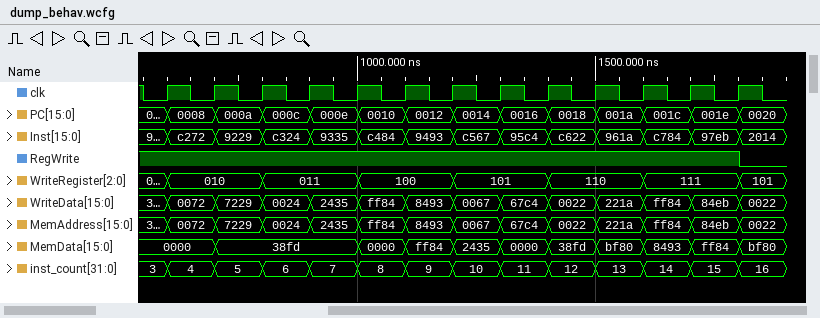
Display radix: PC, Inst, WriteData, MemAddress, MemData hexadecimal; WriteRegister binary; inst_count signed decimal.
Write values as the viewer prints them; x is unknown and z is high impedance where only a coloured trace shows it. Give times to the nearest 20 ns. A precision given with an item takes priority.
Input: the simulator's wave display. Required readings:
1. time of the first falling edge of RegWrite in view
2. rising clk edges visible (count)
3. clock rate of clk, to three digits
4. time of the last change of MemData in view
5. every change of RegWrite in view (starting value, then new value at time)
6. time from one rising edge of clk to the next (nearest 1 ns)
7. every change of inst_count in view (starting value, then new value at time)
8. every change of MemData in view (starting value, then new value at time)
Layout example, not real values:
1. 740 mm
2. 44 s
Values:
1. 1800 ns
2. 13
3. 10.0 MHz
4. 1800 ns
5. 1, 0 at 1800 ns
6. 100 ns
7. 3, 4 at 600 ns, 5 at 700 ns, 6 at 800 ns, 7 at 900 ns, 8 at 1000 ns, 9 at 1100 ns, 10 at 1200 ns, 11 at 1300 ns, 12 at 1400 ns, 13 at 1500 ns, 14 at 1600 ns, 15 at 1700 ns, 16 at 1800 ns
8. 0000, 38fd at 700 ns, 0000 at 1000 ns, ff84 at 1100 ns, 2435 at 1200 ns, 0000 at 1300 ns, 38fd at 1400 ns, bf80 at 1500 ns, 8493 at 1600 ns, ff84 at 1700 ns, bf80 at 1800 ns
